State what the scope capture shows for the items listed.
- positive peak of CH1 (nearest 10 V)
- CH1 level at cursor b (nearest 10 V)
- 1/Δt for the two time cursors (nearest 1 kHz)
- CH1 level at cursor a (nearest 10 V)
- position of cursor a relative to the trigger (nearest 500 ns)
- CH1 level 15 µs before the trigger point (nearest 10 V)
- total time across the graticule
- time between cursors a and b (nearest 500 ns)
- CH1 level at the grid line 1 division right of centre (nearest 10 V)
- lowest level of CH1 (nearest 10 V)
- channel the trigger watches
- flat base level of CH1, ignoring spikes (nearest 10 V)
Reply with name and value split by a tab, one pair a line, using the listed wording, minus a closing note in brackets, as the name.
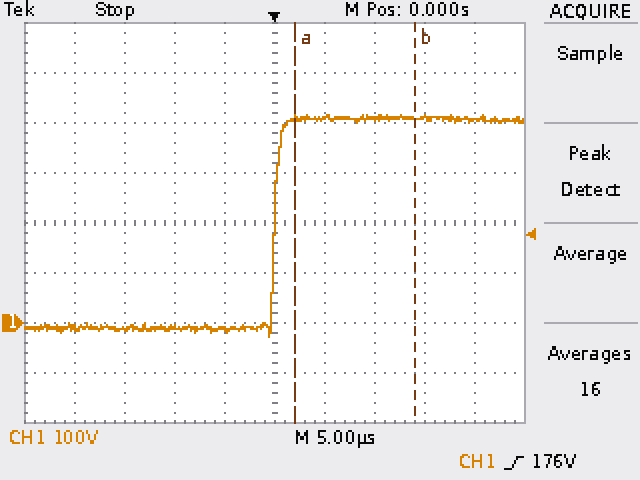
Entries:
positive peak of CH1	420 V
CH1 level at cursor b	410 V
1/Δt for the two time cursors	83 kHz
CH1 level at cursor a	410 V
position of cursor a relative to the trigger	+2.0 µs
CH1 level 15 µs before the trigger point	-10 V
total time across the graticule	50 µs
time between cursors a and b	12.0 µs
CH1 level at the grid line 1 division right of centre	410 V
lowest level of CH1	-30 V
channel the trigger watches	CH1
flat base level of CH1, ignoring spikes	-10 V
